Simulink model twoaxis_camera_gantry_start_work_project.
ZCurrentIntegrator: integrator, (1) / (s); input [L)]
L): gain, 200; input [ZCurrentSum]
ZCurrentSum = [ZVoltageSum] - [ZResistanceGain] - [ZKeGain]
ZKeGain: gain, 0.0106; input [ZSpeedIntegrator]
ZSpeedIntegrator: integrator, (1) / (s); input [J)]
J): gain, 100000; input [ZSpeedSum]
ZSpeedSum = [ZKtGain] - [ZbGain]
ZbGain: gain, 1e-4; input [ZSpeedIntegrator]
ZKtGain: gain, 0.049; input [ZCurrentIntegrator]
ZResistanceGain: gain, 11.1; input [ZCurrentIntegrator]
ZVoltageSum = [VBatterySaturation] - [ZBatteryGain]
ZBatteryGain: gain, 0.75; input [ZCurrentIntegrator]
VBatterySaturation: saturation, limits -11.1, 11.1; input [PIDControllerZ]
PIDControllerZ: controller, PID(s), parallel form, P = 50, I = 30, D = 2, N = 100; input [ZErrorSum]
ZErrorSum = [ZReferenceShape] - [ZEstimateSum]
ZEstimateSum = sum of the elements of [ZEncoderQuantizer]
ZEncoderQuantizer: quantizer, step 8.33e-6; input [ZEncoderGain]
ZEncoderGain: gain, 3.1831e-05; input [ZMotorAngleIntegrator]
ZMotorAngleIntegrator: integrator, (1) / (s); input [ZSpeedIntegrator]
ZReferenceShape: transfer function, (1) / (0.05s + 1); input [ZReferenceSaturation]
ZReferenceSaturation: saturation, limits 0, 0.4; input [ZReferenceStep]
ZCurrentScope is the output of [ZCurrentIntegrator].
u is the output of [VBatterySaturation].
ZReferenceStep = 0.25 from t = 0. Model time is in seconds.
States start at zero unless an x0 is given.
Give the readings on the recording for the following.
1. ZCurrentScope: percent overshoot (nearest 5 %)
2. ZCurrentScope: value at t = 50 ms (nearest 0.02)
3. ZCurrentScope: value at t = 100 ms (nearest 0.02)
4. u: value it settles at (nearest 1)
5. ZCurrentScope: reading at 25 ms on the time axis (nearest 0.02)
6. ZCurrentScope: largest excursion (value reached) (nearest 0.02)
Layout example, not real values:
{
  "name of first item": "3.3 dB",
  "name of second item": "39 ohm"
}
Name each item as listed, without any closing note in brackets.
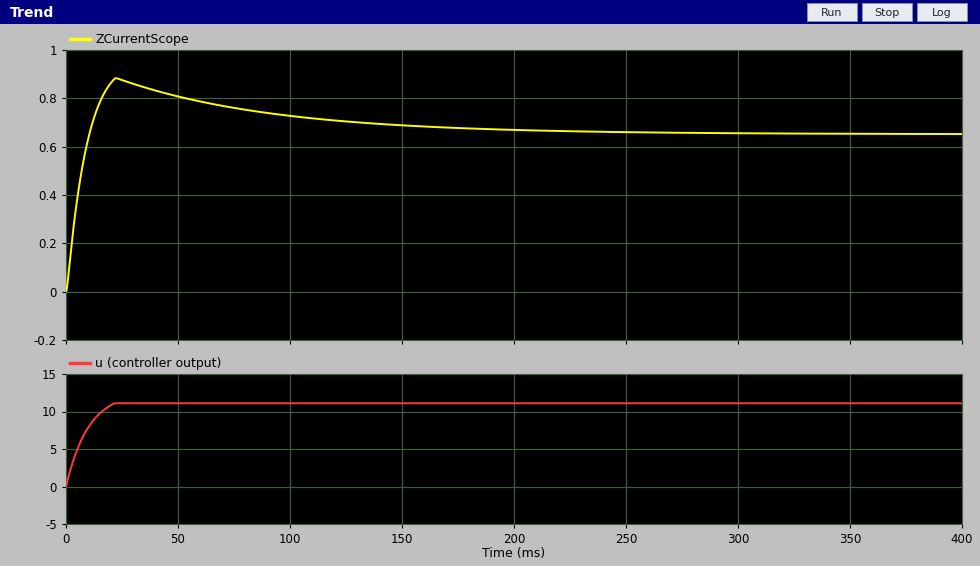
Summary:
{
  "ZCurrentScope: percent overshoot": "35 %",
  "ZCurrentScope: value at t = 50 ms": "0.80",
  "ZCurrentScope: value at t = 100 ms": "0.72",
  "u: value it settles at": "11",
  "ZCurrentScope: reading at 25 ms on the time axis": "0.88",
  "ZCurrentScope: largest excursion (value reached)": "0.88"
}
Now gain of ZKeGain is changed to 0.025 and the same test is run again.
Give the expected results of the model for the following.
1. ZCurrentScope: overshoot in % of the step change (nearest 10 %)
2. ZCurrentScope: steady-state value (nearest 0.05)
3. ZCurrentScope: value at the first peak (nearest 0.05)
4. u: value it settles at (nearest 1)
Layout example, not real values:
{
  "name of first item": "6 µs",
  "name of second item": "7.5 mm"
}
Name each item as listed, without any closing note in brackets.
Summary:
{
  "ZCurrentScope: overshoot in % of the step change": "80 %",
  "ZCurrentScope: steady-state value": "0.45",
  "ZCurrentScope: value at the first peak": "0.80",
  "u: value it settles at": "11"
}
